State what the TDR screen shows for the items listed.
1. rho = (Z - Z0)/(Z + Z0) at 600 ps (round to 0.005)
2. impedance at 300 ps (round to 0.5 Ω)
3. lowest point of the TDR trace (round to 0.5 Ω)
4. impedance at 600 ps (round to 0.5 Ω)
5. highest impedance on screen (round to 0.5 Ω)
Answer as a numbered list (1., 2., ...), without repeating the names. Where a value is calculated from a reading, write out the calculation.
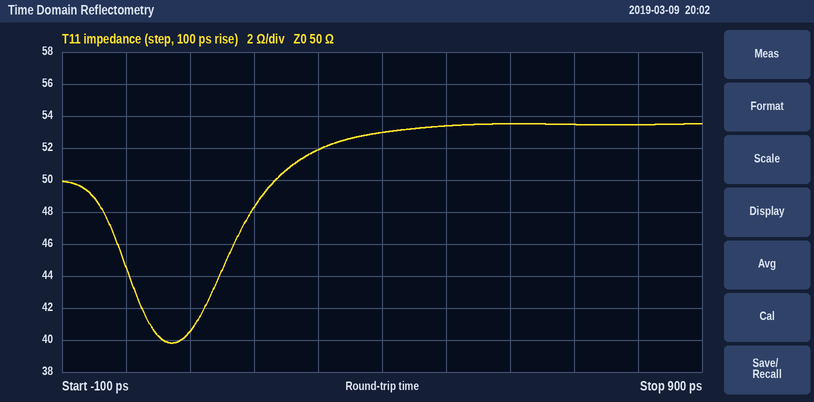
1. (53.5 − 50)/(53.5 + 50) ≈ +0.0338, so +0.035 to the nearest 0.005
2. 52.0 Ω
3. 40.0 Ω
4. 53.5 Ω
5. 53.5 Ω
